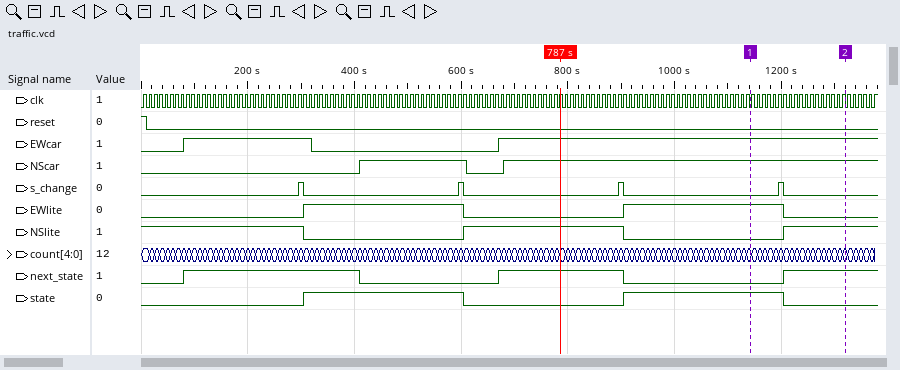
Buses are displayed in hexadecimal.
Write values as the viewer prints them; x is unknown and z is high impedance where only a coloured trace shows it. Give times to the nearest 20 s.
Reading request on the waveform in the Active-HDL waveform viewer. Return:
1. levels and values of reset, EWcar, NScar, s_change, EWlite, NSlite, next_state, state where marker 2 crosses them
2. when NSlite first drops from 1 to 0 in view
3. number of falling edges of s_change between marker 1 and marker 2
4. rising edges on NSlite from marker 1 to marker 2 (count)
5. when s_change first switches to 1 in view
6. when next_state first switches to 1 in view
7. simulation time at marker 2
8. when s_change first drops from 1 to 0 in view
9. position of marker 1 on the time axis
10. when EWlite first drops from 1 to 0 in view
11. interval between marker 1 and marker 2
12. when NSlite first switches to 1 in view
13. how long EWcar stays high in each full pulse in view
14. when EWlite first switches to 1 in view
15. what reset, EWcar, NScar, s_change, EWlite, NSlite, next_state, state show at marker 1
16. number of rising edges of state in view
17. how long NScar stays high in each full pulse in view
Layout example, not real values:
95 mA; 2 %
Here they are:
reset=0, EWcar=1, NScar=1, s_change=0, EWlite=0, NSlite=1, next_state=1, state=0; 300 s; 1; 1; 300 s; 80 s; 1320 s; 300 s; 1140 s; 600 s; 180 s; 600 s; 240 s; 300 s; reset=0, EWcar=1, NScar=1, s_change=0, EWlite=1, NSlite=0, next_state=0, state=1; 2; 200 s
